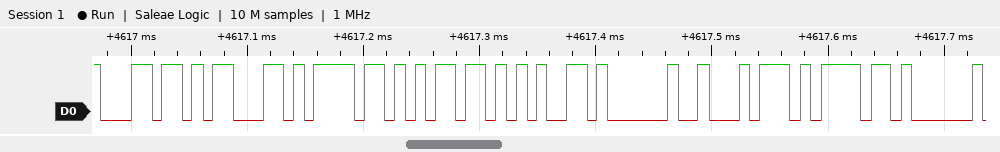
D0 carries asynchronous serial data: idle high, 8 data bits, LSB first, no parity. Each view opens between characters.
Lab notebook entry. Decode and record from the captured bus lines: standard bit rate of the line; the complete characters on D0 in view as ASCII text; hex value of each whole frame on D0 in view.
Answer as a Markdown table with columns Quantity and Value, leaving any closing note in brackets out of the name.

| Quantity | Value |
|---|---|
| standard bit rate of the line | 115200 baud |
| the complete characters on D0 in view as ASCII text | "lcome to" |
| hex value of each whole frame on D0 in view | 6C, 63, 6F, 6D, 65, 20, 74, 6F |
